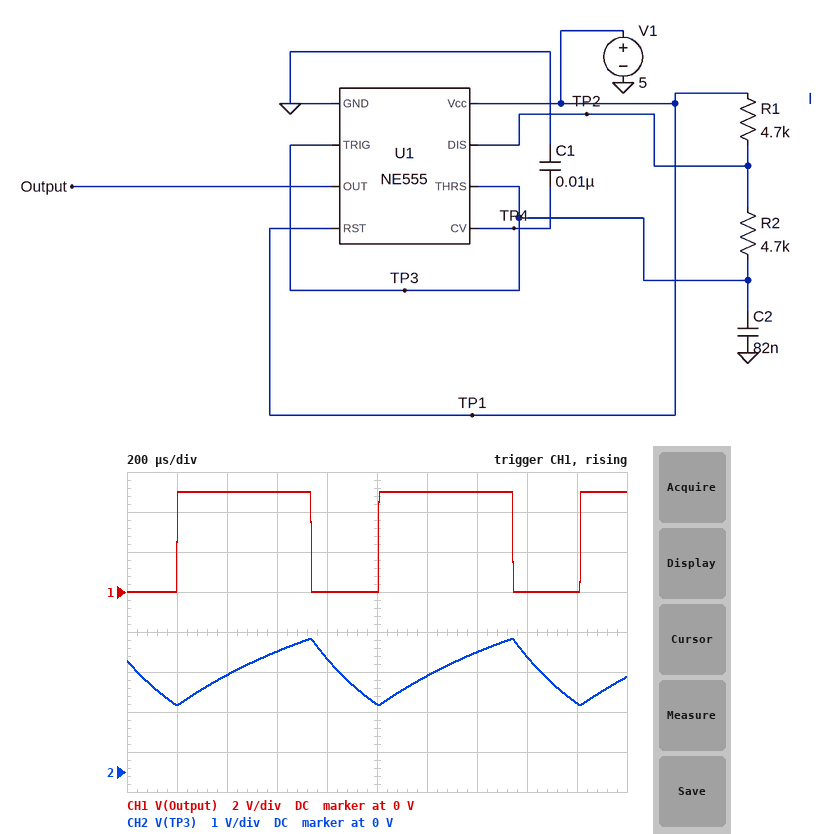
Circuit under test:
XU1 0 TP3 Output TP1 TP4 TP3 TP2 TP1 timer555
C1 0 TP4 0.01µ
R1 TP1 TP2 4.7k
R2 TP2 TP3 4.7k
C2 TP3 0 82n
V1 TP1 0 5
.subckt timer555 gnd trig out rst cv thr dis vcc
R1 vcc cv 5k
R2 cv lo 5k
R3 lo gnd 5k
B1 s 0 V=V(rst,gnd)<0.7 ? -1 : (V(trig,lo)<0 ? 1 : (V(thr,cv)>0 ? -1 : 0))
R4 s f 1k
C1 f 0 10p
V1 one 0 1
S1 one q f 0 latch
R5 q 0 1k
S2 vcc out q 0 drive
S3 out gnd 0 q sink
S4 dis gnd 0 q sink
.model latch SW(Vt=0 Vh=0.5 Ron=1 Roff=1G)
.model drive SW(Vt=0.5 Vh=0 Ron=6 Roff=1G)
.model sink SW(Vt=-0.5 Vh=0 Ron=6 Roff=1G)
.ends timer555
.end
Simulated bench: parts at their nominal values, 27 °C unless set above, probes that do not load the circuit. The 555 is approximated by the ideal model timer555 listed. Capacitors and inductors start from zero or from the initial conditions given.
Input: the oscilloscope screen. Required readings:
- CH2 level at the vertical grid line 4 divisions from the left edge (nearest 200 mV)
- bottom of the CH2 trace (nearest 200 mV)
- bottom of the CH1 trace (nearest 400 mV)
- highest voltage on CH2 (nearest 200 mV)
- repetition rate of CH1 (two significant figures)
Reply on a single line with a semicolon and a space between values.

2.8 V; 1.6 V; 0 V; 3.4 V; 1.2 kHz
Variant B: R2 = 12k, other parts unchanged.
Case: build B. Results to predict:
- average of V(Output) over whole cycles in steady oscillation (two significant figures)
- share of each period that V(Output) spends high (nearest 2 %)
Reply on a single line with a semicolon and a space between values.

2.9 V; 58 %
